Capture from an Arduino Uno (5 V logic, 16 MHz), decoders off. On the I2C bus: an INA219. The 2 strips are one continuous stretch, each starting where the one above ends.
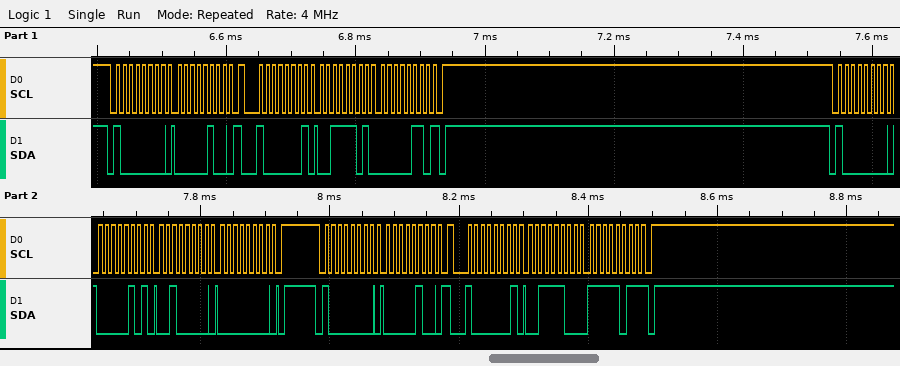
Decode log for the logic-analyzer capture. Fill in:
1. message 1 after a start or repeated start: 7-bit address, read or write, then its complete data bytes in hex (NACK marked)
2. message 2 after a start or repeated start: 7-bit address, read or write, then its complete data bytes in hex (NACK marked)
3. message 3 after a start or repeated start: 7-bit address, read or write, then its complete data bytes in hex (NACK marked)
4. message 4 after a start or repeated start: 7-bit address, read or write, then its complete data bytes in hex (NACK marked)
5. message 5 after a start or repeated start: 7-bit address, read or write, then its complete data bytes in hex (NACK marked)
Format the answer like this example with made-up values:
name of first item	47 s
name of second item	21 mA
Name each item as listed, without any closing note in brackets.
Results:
message 1 after a start or repeated start: 7-bit address, read or write, then its complete data bytes in hex	0x40 write: 04
message 2 after a start or repeated start: 7-bit address, read or write, then its complete data bytes in hex	0x40 read: 3D 06 NACK
message 3 after a start or repeated start: 7-bit address, read or write, then its complete data bytes in hex	0x40 write: 05 20 00
message 4 after a start or repeated start: 7-bit address, read or write, then its complete data bytes in hex	0x40 write: 04
message 5 after a start or repeated start: 7-bit address, read or write, then its complete data bytes in hex	0x40 read: 3C FB NACK
